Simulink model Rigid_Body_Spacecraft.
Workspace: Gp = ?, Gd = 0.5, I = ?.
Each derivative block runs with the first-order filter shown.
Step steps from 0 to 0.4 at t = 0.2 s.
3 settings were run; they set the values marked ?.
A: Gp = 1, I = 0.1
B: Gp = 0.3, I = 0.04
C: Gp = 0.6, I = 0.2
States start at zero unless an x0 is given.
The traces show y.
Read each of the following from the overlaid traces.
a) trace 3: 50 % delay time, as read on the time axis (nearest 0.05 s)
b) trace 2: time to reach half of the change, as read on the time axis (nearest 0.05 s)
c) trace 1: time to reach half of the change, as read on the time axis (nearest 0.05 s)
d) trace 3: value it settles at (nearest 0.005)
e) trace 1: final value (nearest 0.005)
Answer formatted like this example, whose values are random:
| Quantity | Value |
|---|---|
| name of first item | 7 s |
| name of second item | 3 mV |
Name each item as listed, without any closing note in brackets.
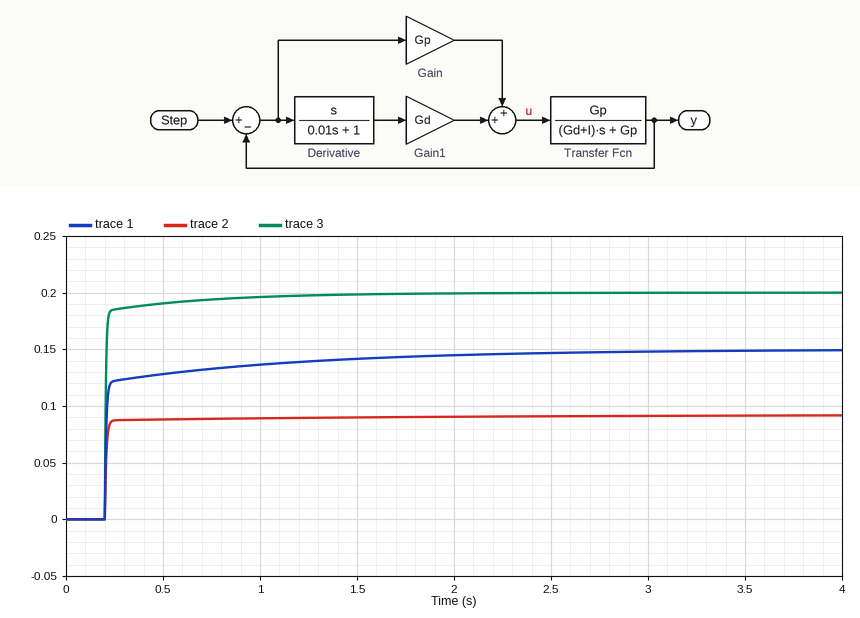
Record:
| Quantity | Value |
|---|---|
| trace 3: 50 % delay time, as read on the time axis | 0.20 s |
| trace 2: time to reach half of the change, as read on the time axis | 0.20 s |
| trace 1: time to reach half of the change, as read on the time axis | 0.20 s |
| trace 3: value it settles at | 0.200 |
| trace 1: final value | 0.150 |
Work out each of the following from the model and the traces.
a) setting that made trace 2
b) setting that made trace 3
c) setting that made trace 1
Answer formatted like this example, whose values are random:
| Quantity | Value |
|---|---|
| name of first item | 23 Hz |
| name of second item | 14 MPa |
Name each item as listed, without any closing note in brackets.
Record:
| Quantity | Value |
|---|---|
| setting that made trace 2 | B |
| setting that made trace 3 | A |
| setting that made trace 1 | C |
